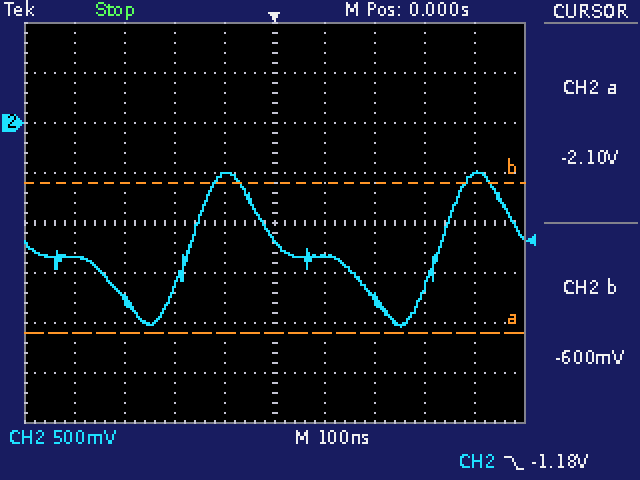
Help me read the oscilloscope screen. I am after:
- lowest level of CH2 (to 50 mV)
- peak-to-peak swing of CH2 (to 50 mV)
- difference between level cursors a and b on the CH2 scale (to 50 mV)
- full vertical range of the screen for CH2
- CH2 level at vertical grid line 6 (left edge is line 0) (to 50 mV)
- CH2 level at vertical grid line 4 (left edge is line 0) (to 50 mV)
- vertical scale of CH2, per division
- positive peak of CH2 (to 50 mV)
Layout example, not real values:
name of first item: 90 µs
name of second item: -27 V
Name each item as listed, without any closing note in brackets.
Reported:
lowest level of CH2: -2.05 V
peak-to-peak swing of CH2: 1.55 V
difference between level cursors a and b on the CH2 scale: 1.50 V
full vertical range of the screen for CH2: 4 V
CH2 level at vertical grid line 6 (left edge is line 0): -1.35 V
CH2 level at vertical grid line 4 (left edge is line 0): -500 mV
vertical scale of CH2, per division: 500 mV
positive peak of CH2: -500 mV
